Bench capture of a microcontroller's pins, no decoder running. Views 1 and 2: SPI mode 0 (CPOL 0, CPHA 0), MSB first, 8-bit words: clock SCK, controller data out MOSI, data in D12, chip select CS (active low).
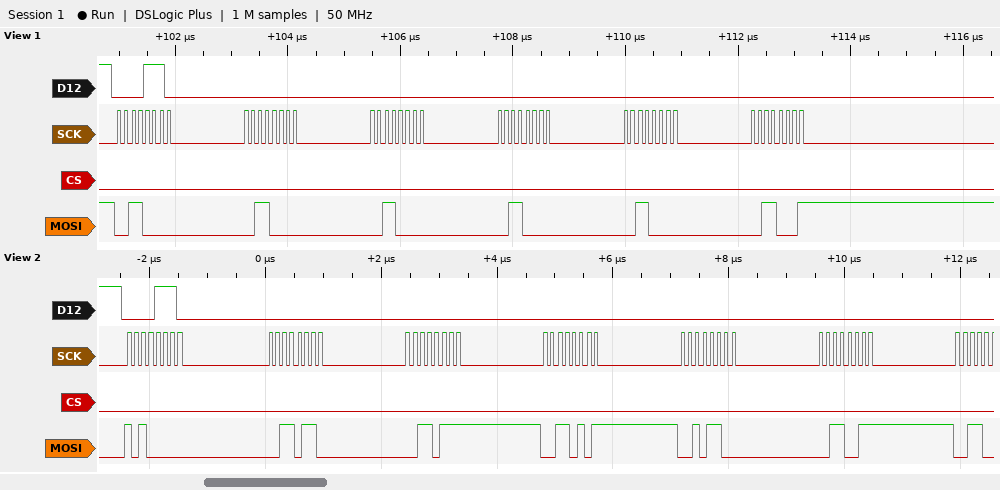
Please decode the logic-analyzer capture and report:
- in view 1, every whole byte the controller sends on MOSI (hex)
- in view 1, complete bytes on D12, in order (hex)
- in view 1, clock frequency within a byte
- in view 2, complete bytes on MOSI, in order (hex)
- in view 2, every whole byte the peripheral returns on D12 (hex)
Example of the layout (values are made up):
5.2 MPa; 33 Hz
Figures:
0x30 0x30 0x30 0x30 0x30 0x31; 0x0E 0x00 0x00 0x00 0x00 0x00; 8 MHz; 0xA0 0x36 0x37 0x35 0x2C 0x33; 0x0E 0x00 0x00 0x00 0x00 0x00
